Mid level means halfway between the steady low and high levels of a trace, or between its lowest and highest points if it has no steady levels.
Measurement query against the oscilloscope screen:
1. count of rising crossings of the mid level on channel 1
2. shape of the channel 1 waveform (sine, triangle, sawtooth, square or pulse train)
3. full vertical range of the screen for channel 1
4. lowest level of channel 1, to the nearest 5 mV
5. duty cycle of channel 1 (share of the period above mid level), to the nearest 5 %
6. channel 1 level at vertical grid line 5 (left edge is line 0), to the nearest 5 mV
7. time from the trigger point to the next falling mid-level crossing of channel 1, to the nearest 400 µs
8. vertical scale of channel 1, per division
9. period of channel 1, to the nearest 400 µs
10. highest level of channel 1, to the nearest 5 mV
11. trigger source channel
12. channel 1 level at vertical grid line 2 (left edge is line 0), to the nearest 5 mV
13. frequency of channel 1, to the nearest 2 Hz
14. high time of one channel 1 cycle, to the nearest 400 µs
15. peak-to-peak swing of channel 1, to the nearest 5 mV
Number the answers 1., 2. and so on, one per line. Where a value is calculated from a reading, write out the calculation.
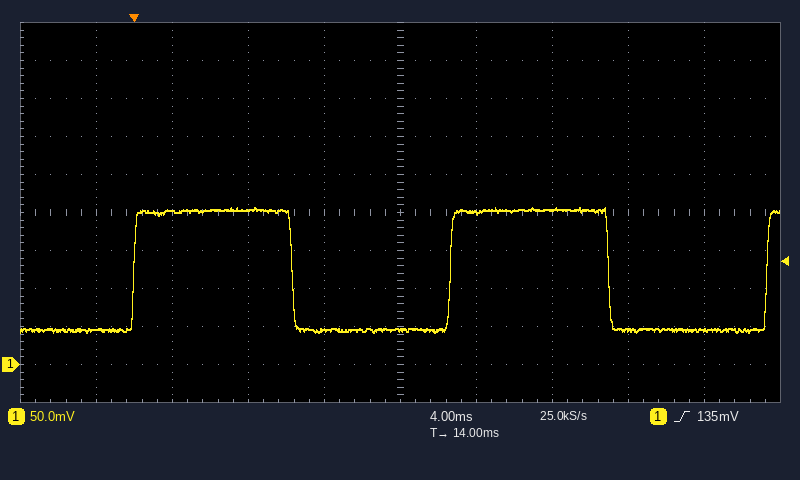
1. 3
2. square
3. 500 mV
4. 40 mV
5. 8.4 ms / 16.8 ms ≈ 50 %
6. 45 mV
7. 8.4 ms
8. 50 mV
9. 16.8 ms
10. 205 mV
11. channel 1
12. 200 mV
13. 1 / 16.8 ms ≈ 60 Hz
14. 8.4 ms
15. 205 mV − (40 mV) = 165 mV
